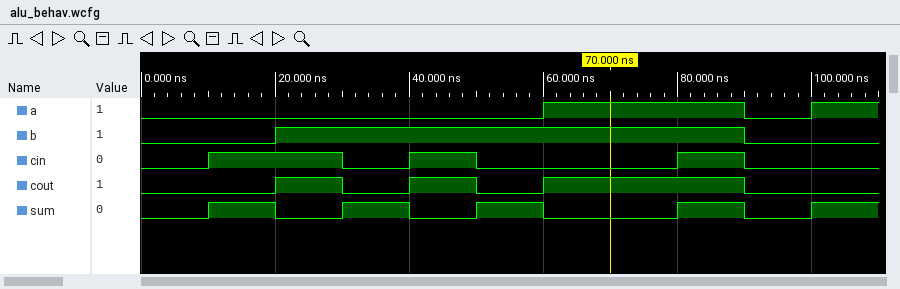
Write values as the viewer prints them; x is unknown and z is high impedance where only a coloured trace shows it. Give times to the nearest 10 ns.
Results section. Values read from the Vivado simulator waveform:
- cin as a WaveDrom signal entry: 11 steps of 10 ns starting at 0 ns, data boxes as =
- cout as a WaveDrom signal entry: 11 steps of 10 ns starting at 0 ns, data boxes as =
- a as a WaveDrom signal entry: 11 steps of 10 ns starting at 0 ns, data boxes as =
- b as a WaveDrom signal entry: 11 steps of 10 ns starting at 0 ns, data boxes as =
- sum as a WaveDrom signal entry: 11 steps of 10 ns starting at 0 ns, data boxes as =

{name: 'cin', wave: '01.010..10.'}
{name: 'cout', wave: '0.10101..0.'}
{name: 'a', wave: '0.....1..01'}
{name: 'b', wave: '0.1......0.'}
{name: 'sum', wave: '0101010.101'}
